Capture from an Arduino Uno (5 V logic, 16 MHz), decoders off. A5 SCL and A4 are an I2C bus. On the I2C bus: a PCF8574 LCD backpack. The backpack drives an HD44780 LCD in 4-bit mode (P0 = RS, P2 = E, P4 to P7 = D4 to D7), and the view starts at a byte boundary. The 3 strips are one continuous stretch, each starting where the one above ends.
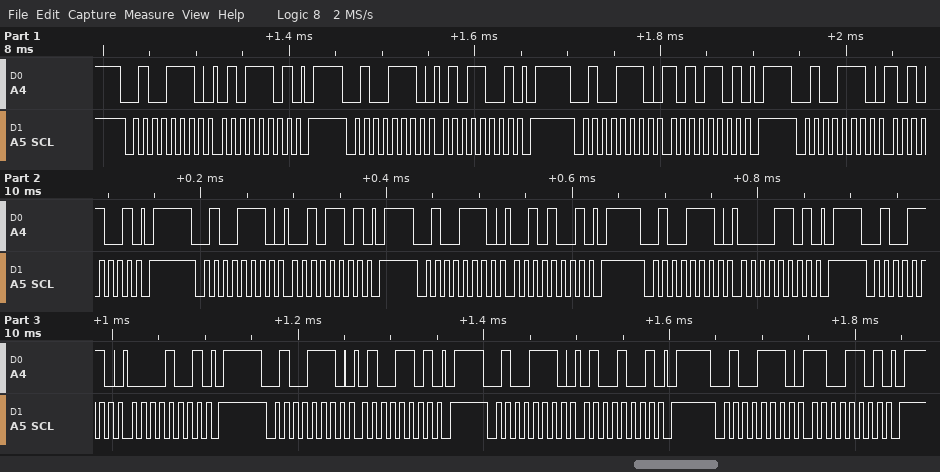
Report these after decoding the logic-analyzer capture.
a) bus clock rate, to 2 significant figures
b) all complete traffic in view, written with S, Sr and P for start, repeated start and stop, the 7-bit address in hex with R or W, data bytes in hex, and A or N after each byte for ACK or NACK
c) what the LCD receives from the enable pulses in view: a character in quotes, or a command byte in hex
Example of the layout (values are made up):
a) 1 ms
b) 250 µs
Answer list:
a) 100 kHz
b) S 27W A 5D A P S 27W A 59 A P S 27W A AD A P S 27W A A9 A P S 27W A 2D A P S 27W A 29 A P S 27W A 0D A P S 27W A 09 A P S 27W A 4D A P S 27W A 49 A P S 27W A CD A P
c) 'Z' ' '
